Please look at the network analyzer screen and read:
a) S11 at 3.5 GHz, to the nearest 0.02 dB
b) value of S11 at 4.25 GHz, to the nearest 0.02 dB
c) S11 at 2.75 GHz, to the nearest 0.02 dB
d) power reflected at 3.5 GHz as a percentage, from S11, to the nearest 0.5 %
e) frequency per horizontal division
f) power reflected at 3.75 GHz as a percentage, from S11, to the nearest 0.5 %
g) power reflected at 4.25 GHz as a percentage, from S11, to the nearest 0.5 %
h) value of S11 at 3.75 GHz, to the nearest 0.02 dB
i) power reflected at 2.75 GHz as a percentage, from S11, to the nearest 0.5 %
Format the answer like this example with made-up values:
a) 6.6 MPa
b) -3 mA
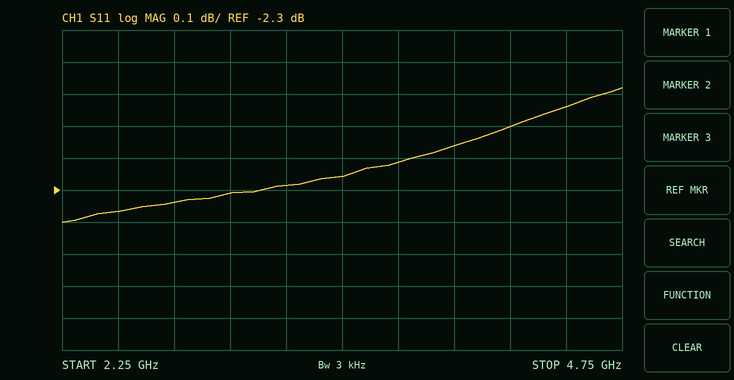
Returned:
a) -2.26 dB
b) -2.10 dB
c) -2.34 dB
d) 59.5 %
e) 250 MHz
f) 60.0 %
g) 61.5 %
h) -2.22 dB
i) 58.5 %
